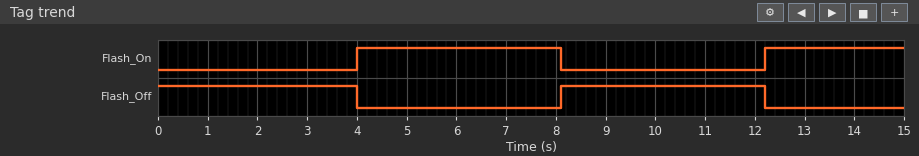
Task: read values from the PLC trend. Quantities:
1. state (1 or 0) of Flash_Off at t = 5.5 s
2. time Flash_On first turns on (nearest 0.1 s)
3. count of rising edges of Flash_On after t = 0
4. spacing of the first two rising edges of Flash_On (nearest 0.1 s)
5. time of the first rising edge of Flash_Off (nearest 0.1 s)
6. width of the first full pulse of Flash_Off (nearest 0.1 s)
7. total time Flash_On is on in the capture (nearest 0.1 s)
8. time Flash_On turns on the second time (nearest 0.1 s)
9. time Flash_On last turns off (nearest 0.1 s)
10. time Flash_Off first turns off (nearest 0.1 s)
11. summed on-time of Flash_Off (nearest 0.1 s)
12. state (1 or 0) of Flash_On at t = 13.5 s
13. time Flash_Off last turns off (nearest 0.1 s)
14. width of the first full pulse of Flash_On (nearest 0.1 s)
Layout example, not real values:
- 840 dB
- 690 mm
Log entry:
- 0
- 4.0 s
- 2
- 8.2 s
- 8.1 s
- 4.1 s
- 6.9 s
- 12.2 s
- 8.1 s
- 4.0 s
- 8.1 s
- 1
- 12.2 s
- 4.1 s
